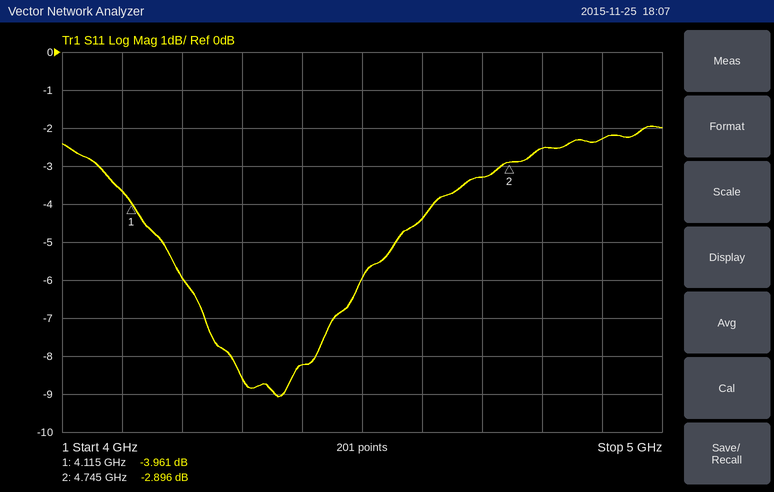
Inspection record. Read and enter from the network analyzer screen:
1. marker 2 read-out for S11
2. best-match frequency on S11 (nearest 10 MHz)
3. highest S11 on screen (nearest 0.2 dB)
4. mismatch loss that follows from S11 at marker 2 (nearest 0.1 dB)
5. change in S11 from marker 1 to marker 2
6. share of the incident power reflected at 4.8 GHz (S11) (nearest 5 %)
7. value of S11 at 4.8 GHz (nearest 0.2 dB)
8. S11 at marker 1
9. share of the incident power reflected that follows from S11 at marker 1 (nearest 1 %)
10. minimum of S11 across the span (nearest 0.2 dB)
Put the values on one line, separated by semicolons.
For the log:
-2.896 dB; 4.36 GHz; -2.0 dB; 3.1 dB; 1.065 dB; 55 %; -2.6 dB; -3.961 dB; 40 %; -9.0 dB
